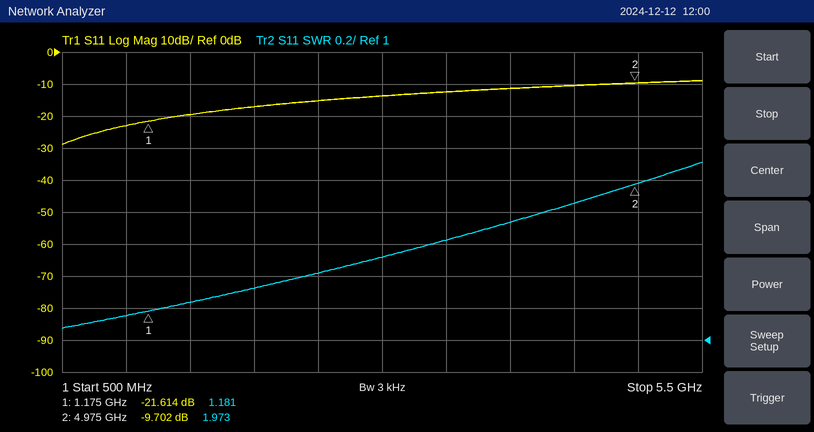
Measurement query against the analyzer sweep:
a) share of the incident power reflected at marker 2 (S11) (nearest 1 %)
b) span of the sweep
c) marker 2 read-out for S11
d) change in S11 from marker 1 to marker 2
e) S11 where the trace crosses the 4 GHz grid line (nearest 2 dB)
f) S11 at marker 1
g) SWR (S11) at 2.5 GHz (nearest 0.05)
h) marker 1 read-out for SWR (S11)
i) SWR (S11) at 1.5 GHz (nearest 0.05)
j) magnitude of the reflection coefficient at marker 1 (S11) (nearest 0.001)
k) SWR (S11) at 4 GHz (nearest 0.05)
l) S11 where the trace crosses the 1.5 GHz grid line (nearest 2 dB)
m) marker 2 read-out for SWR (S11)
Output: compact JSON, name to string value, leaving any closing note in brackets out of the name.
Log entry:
{"share of the incident power reflected at marker 2 (S11)": "11 %", "span of the sweep": "5 GHz", "marker 2 read-out for S11": "-9.702 dB", "change in S11 from marker 1 to marker 2": "11.912 dB", "S11 where the trace crosses the 4 GHz grid line": "-12 dB", "S11 at marker 1": "-21.614 dB", "SWR (S11) at 2.5 GHz": "1.40", "marker 1 read-out for SWR": "1.181", "SWR (S11) at 1.5 GHz": "1.25", "magnitude of the reflection coefficient at marker 1 (S11)": "0.083", "SWR (S11) at 4 GHz": "1.75", "S11 where the trace crosses the 1.5 GHz grid line": "-20 dB", "marker 2 read-out for SWR": "1.973"}
